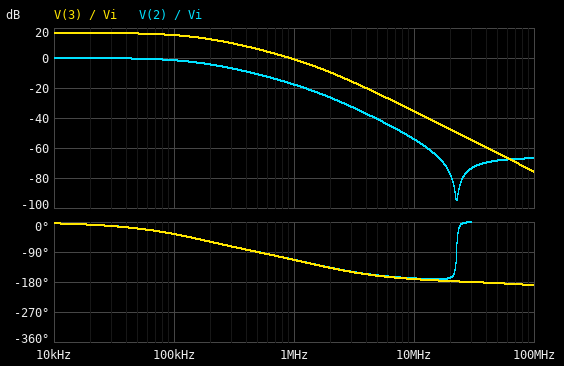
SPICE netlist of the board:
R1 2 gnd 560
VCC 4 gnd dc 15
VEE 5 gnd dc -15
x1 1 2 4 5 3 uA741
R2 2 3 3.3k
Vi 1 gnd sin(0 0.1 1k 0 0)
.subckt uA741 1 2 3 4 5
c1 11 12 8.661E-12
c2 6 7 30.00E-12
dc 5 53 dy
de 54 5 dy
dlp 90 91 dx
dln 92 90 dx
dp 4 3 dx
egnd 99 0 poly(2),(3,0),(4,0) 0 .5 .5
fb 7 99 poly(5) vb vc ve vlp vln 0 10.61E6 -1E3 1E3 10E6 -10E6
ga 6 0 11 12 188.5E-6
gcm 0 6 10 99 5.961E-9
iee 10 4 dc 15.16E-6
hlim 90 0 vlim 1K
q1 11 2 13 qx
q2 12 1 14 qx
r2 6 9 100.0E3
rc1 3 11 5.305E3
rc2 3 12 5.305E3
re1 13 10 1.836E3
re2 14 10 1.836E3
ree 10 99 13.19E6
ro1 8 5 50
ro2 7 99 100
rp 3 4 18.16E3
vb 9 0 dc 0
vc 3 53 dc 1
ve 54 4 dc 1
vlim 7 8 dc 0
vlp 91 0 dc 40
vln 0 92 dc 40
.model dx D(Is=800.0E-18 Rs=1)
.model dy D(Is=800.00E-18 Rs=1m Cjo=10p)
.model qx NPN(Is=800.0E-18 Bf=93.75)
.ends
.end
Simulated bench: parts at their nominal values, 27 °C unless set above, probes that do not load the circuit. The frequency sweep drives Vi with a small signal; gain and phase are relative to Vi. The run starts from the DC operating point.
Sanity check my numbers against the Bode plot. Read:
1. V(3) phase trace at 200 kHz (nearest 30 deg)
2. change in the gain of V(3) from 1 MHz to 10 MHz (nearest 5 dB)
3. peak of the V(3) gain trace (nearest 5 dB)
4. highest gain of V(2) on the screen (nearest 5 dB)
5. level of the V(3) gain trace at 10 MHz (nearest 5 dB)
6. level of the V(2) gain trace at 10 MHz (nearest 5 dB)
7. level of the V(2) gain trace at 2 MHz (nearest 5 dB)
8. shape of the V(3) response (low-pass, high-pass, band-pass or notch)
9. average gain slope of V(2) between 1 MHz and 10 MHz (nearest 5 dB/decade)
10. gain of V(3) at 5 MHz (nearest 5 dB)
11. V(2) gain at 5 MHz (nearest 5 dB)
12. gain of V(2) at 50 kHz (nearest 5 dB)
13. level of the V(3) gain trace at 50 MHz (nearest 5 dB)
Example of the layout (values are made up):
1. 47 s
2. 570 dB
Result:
1. -60 deg
2. -35 dB
3. 15 dB
4. 0 dB
5. -35 dB
6. -55 dB
7. -25 dB
8. low-pass
9. -35 dB/decade
10. -25 dB
11. -40 dB
12. 0 dB
13. -65 dB
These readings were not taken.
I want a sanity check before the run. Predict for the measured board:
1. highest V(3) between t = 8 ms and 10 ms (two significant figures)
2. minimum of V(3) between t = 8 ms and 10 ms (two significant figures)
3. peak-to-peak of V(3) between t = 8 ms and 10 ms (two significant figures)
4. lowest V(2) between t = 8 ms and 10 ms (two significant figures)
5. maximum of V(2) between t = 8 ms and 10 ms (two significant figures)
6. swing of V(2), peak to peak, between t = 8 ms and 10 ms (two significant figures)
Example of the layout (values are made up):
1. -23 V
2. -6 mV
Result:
1. 690 mV
2. -690 mV
3. 1.4 V
4. -100 mV
5. 100 mV
6. 200 mV
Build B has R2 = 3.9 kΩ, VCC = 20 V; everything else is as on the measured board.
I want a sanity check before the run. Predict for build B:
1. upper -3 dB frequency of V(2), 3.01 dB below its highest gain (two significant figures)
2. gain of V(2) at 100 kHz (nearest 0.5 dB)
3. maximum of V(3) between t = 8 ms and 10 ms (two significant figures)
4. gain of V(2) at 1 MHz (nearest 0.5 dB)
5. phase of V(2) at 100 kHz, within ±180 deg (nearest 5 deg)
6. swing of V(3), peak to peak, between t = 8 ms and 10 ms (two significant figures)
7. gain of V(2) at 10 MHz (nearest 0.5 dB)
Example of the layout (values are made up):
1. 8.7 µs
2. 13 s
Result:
1. 130 kHz
2. -2.0 dB
3. 800 mV
4. -19.0 dB
5. -40 deg
6. 1.6 V
7. -56.0 dB
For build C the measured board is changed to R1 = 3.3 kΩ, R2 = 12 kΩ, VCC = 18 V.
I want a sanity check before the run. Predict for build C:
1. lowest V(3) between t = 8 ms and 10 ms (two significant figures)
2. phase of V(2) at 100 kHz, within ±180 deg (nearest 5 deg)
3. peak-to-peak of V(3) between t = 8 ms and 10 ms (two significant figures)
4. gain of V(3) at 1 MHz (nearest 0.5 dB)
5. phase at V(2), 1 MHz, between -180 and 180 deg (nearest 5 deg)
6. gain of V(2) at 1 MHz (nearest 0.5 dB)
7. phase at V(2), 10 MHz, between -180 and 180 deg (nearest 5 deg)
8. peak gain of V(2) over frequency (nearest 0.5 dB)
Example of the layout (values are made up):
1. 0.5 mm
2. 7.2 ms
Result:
1. -460 mV
2. -25 deg
3. 930 mV
4. -0.5 dB
5. -110 deg
6. -14.0 dB
7. -150 deg
8. 0 dB
